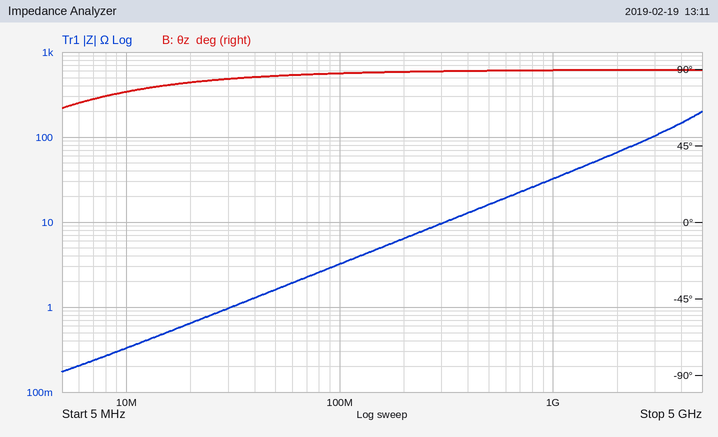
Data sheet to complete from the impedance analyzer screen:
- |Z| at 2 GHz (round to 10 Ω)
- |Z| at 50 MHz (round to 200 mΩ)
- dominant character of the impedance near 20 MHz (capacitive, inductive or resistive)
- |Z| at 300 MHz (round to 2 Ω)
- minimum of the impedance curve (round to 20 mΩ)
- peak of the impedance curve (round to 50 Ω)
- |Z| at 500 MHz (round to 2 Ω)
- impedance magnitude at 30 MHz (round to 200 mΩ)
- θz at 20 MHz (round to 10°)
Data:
70 Ω
1.6 Ω
inductive
10 Ω
180 mΩ
200 Ω
16 Ω
1.0 Ω
80°
